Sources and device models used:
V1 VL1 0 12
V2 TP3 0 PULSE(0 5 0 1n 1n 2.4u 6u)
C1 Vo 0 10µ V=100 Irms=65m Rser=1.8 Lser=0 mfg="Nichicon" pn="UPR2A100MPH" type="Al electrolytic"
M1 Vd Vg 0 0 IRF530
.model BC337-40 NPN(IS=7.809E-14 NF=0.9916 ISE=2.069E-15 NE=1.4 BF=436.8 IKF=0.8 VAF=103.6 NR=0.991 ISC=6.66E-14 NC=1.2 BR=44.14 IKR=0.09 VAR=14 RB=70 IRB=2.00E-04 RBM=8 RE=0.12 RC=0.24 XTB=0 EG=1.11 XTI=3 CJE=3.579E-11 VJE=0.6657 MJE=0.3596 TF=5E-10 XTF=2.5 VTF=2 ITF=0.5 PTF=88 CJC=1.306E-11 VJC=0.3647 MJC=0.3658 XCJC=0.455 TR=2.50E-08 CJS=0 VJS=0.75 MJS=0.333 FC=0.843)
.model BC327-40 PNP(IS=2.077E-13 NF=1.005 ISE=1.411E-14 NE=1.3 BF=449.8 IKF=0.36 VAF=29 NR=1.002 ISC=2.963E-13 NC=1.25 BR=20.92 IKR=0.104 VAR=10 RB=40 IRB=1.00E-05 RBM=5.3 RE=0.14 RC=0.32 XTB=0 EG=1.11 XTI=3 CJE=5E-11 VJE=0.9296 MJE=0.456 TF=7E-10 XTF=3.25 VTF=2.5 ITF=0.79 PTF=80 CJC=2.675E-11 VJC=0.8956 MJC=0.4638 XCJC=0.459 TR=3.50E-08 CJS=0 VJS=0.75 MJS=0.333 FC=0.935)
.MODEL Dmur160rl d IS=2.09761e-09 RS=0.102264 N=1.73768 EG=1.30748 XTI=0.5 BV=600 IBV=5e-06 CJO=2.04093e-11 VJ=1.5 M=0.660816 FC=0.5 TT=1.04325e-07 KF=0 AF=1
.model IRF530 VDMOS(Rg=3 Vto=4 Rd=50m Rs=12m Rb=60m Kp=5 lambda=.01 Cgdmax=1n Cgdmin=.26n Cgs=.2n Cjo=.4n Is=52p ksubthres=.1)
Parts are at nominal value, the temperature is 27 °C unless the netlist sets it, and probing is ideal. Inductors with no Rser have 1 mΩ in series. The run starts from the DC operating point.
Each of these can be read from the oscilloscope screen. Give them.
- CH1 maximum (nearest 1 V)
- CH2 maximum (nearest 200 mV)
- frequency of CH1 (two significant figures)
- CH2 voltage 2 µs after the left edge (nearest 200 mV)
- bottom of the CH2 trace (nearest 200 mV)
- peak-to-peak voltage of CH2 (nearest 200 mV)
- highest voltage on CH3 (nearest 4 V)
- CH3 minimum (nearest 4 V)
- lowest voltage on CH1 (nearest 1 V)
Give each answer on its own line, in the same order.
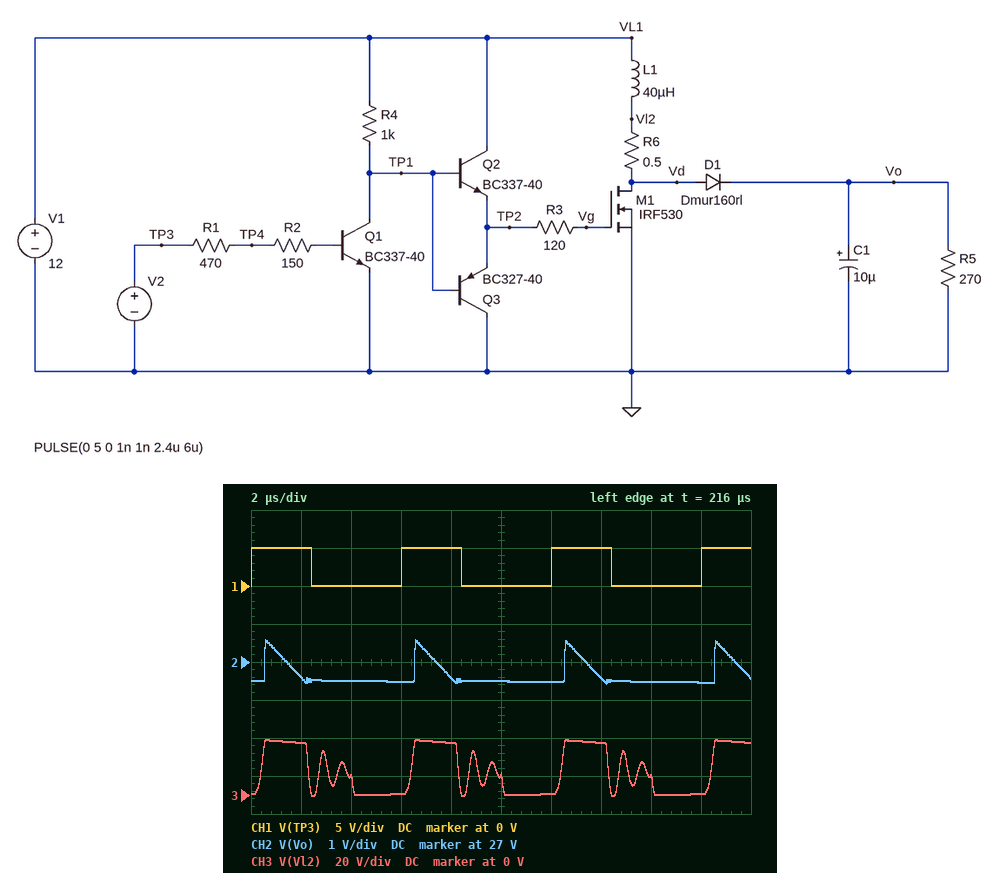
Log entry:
5 V
27.6 V
170 kHz
26.6 V
26.4 V
1.2 V
28 V
0 V
0 V
